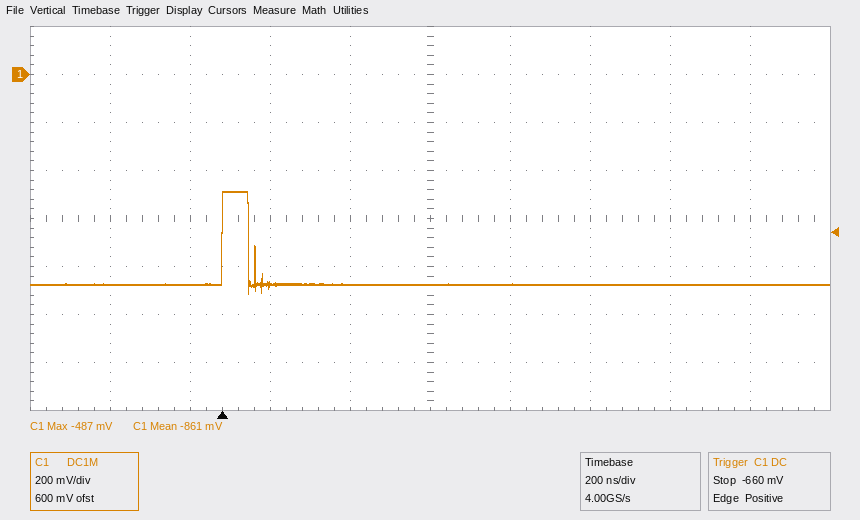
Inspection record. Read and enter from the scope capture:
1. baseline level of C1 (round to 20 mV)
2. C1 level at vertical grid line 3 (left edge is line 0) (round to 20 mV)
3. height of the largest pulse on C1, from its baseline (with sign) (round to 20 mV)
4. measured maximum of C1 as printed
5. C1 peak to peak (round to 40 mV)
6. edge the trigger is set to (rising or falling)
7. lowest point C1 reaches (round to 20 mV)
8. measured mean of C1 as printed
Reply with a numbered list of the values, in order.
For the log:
1. -880 mV
2. -880 mV
3. +380 mV
4. -487 mV
5. 440 mV
6. rising
7. -920 mV
8. -861 mV
